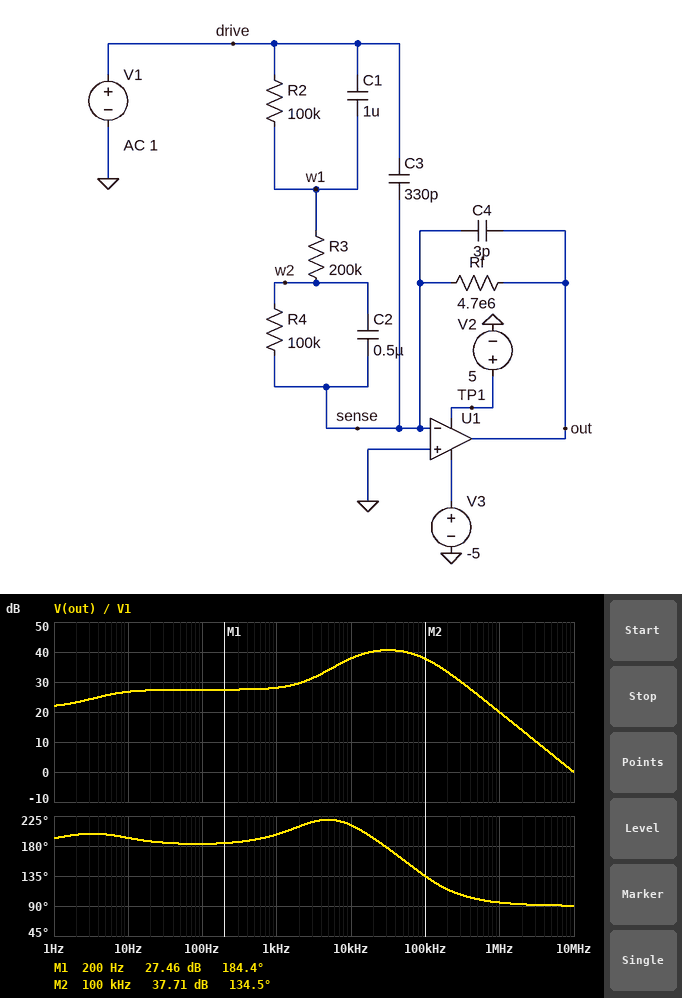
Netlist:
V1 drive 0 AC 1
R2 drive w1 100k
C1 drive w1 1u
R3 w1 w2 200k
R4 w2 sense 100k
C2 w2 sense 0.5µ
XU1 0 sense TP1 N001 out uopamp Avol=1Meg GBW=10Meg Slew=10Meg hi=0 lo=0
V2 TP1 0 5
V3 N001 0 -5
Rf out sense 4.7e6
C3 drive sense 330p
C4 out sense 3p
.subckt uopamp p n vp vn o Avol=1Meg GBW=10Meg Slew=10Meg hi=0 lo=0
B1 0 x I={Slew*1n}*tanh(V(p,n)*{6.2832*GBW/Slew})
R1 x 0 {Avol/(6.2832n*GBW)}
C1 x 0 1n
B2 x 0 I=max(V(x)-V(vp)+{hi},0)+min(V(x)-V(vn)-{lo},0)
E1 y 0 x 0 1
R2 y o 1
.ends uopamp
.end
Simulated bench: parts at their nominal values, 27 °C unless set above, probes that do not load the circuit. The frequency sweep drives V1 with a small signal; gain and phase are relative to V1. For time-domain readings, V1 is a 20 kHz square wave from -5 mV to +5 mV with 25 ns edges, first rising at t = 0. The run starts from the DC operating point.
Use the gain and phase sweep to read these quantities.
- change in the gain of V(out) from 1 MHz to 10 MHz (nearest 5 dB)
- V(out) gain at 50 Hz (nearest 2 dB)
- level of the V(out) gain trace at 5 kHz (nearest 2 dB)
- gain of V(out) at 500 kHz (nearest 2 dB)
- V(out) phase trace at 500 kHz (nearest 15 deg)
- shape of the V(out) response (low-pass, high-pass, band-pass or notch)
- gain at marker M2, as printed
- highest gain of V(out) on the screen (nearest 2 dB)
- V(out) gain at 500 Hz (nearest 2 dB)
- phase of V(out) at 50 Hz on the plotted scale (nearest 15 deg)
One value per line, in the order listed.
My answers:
-20 dB
28 dB
34 dB
26 dB
105 deg
band-pass
37.71 dB
40 dB
28 dB
180 deg
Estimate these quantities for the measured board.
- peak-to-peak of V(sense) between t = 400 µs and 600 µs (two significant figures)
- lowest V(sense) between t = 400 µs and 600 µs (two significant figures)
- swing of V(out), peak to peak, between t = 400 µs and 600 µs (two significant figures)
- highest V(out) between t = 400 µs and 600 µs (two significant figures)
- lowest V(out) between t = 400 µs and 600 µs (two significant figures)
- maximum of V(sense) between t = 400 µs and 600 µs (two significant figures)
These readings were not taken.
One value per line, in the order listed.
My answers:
20 mV
-10 mV
1.4 V
650 mV
-770 mV
10 mV
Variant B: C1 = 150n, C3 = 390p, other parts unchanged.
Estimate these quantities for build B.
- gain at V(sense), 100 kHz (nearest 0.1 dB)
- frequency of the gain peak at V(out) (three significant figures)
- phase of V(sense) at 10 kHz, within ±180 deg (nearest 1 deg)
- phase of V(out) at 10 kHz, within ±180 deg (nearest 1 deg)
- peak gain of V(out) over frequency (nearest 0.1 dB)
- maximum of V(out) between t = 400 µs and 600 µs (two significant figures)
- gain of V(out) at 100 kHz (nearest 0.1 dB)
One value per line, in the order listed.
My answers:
-1.7 dB
29.1 kHz
123 deg
-147 deg
42.1 dB
780 mV
38.3 dB
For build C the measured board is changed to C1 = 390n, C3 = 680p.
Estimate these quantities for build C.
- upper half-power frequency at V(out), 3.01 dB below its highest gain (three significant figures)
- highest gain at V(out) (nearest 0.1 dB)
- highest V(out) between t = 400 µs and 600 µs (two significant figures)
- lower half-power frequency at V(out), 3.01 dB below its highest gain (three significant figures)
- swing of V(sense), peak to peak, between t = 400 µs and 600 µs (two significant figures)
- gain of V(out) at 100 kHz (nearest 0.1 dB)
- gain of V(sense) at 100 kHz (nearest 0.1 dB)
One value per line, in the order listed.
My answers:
54.2 kHz
46.9 dB
1.3 V
9.04 kHz
21 mV
39.5 dB
-0.5 dB
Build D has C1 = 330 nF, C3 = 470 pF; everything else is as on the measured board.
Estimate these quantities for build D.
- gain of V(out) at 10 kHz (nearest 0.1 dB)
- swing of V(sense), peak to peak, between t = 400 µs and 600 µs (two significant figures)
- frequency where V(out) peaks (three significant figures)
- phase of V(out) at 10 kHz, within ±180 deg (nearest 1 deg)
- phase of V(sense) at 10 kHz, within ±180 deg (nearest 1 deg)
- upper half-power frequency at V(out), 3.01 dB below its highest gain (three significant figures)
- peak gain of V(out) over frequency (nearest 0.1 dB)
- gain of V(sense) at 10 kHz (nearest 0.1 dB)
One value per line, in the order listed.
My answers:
41.0 dB
20 mV
26.6 kHz
-146 deg
124 deg
74.6 kHz
43.7 dB
-19.0 dB
